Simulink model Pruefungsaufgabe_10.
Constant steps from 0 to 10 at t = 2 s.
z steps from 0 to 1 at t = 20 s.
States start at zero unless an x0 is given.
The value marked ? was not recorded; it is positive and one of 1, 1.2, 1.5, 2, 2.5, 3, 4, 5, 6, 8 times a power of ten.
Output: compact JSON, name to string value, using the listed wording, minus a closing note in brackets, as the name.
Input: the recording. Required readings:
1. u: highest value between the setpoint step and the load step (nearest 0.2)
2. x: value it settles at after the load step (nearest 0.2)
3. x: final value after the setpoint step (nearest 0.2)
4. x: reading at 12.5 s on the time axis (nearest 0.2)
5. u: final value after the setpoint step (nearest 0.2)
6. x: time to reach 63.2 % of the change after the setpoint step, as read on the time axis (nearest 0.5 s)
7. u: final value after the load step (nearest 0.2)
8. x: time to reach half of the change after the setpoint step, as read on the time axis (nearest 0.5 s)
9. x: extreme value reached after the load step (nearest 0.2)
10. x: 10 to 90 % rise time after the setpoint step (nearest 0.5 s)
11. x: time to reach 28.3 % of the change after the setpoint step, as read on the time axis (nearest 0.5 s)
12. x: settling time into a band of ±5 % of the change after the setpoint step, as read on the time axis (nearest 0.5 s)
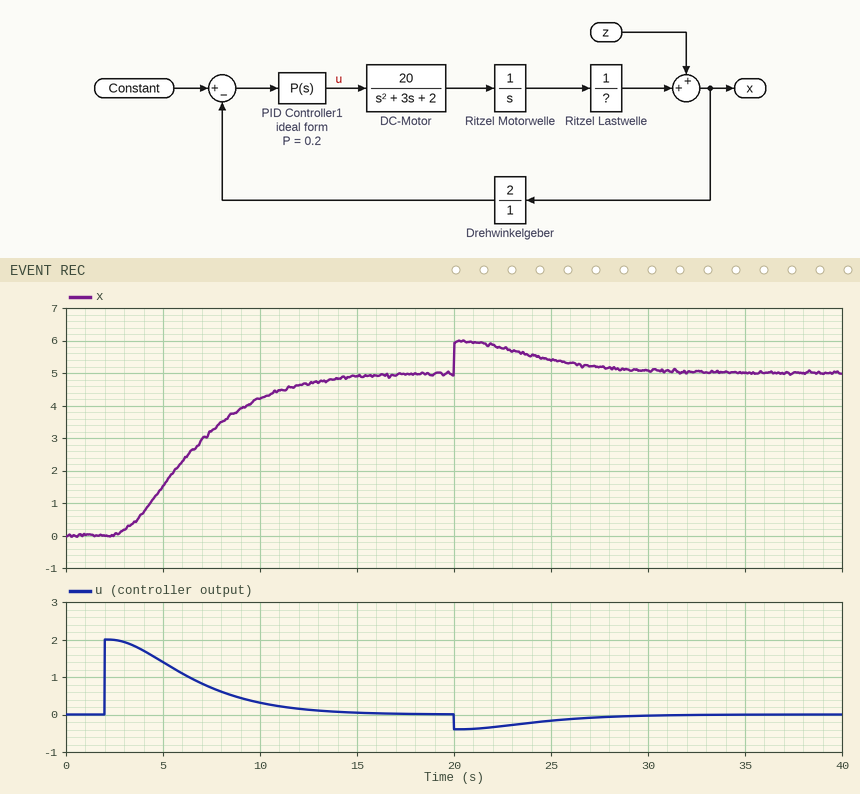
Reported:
{"u: highest value between the setpoint step and the load step": "2.0", "x: value it settles at after the load step": "5.0", "x: final value after the setpoint step": "5.0", "x: reading at 12.5 s on the time axis": "4.6", "u: final value after the setpoint step": "0.0", "x: time to reach 63.2 % of the change after the setpoint step, as read on the time axis": "7.5 s", "u: final value after the load step": "0.0", "x: time to reach half of the change after the setpoint step, as read on the time axis": "6.5 s", "x: extreme value reached after the load step": "6.0", "x: 10 to 90 % rise time after the setpoint step": "7.5 s", "x: time to reach 28.3 % of the change after the setpoint step, as read on the time axis": "5.0 s", "x: settling time into a band of ±5 % of the change after the setpoint step, as read on the time axis": "13.0 s"}
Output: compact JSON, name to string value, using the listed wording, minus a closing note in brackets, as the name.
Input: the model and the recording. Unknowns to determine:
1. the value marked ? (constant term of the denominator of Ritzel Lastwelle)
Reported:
{"the value marked ?": "20"}
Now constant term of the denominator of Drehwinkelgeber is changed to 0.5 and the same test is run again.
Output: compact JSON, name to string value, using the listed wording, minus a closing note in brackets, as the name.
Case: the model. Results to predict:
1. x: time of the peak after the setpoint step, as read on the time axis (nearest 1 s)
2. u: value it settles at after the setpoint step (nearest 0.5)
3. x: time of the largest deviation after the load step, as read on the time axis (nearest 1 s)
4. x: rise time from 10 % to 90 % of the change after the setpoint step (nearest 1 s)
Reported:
{"x: time of the peak after the setpoint step, as read on the time axis": "9 s", "u: value it settles at after the setpoint step": "0.0", "x: time of the largest deviation after the load step, as read on the time axis": "20 s", "x: rise time from 10 % to 90 % of the change after the setpoint step": "3 s"}
